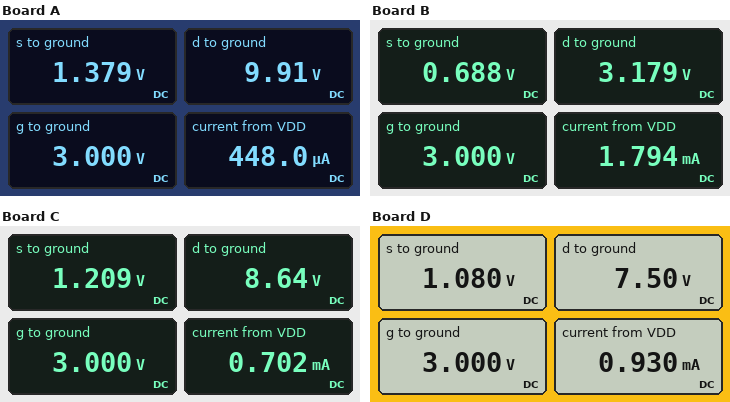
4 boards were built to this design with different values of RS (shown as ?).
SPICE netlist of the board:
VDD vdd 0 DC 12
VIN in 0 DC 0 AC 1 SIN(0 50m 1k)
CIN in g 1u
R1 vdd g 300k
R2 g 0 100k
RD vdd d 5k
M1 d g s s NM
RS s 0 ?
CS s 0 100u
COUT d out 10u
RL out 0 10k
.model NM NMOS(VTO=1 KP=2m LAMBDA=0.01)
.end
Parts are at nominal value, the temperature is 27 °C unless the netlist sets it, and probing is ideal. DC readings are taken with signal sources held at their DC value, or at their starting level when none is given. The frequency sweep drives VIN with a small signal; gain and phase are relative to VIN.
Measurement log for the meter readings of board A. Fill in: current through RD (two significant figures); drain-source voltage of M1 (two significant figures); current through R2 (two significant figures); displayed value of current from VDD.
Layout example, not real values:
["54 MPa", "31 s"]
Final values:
["420 µA", "8.5 V", "30 µA", "448.0 µA"]
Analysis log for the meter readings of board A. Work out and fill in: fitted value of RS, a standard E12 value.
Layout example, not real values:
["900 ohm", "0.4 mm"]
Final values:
["3.3 kΩ"]
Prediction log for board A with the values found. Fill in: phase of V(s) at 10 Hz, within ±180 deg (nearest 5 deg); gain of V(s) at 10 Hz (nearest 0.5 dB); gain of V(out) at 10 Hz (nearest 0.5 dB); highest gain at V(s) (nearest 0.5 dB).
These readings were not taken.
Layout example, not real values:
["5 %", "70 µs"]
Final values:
["-65 deg", "-14.0 dB", "12.5 dB", "-7.0 dB"]
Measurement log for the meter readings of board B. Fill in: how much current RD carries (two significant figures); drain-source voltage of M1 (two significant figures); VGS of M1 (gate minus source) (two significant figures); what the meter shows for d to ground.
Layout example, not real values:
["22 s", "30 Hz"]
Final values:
["1.8 mA", "2.5 V", "2.3 V", "3.179 V"]
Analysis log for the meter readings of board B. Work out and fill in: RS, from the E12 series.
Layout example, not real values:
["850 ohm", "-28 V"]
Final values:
["390 Ω"]
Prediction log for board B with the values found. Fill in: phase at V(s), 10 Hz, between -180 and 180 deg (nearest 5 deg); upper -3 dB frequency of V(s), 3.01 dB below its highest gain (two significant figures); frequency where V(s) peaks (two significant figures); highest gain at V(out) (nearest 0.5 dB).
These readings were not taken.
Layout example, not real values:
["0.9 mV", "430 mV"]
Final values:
["-40 deg", "12 Hz", "4.2 Hz", "18.5 dB"]
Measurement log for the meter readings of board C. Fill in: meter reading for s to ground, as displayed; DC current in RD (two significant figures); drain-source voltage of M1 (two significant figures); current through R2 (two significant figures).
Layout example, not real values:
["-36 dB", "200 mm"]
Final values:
["1.209 V", "670 µA", "7.4 V", "30 µA"]
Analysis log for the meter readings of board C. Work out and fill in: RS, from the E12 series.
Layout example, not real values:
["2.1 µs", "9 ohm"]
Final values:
["1.8 kΩ"]
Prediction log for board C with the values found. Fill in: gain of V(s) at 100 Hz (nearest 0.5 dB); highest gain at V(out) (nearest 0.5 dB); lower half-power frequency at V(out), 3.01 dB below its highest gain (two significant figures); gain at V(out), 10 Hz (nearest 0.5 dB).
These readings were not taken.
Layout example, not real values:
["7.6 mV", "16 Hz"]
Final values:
["-31.5 dB", "15.0 dB", "4.5 Hz", "14.0 dB"]
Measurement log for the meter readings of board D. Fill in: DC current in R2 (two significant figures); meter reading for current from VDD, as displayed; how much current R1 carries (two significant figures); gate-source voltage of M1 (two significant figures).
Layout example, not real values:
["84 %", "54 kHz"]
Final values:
["30 µA", "0.930 mA", "30 µA", "1.9 V"]
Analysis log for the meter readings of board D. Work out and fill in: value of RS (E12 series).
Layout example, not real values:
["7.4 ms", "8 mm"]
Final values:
["1.2 kΩ"]
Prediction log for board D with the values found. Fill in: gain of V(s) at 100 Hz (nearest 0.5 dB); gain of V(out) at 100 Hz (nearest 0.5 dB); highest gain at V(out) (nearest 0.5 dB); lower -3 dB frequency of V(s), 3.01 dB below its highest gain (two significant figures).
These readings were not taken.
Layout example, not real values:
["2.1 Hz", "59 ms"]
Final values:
["-30.5 dB", "16.0 dB", "16.0 dB", "1.2 Hz"]
